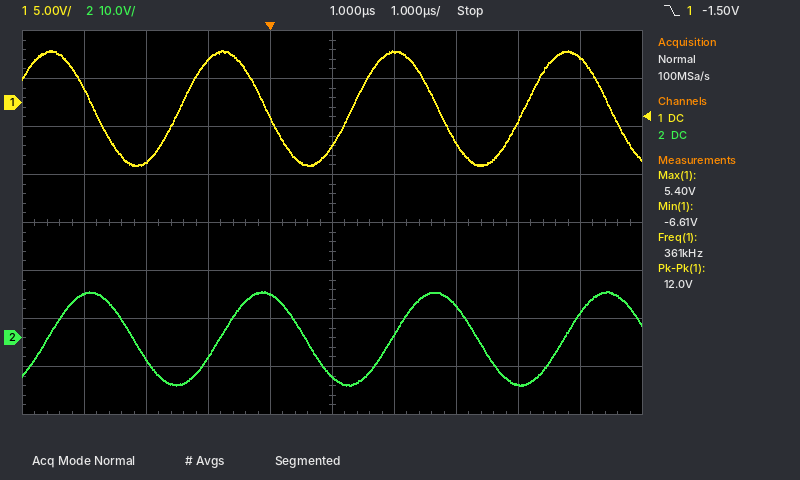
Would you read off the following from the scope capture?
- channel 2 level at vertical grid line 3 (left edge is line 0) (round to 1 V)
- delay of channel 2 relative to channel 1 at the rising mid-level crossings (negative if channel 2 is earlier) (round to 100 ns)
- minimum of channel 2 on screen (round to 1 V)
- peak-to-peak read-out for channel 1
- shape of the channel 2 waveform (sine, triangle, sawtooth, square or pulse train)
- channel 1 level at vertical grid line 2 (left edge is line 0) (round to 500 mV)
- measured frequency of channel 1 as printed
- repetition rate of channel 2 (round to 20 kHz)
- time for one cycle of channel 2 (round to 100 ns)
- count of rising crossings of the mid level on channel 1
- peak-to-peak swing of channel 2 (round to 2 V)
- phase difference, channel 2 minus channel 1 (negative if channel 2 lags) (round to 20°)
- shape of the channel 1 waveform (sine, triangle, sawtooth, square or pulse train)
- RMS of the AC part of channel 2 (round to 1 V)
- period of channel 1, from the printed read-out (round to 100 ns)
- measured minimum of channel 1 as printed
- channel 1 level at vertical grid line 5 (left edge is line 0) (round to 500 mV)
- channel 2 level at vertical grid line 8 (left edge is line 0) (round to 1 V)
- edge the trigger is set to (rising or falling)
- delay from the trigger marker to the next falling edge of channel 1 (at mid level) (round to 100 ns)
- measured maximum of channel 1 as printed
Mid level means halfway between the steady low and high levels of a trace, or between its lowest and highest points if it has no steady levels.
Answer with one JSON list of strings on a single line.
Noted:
["-4 V", "+600 ns", "-10 V", "12.0 V", "sine", "-6.0 V", "361 kHz", "360 kHz", "2.8 µs", "3", "20 V", "-80°", "sine", "7 V", "2.8 µs", "-6.61 V", "-4.5 V", "-10 V", "falling", "2.7 µs", "5.40 V"]
